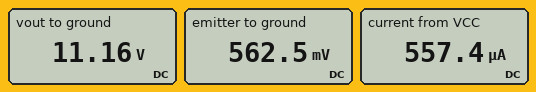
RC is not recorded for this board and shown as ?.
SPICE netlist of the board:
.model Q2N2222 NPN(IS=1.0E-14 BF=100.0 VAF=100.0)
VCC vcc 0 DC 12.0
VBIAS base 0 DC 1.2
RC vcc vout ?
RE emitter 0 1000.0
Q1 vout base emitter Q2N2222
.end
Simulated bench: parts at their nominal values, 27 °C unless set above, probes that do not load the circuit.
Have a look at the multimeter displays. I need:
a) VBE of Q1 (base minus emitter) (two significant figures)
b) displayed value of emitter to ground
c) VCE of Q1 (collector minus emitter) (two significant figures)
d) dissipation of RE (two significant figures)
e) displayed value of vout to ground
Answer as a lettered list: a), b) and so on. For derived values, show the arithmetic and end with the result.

a) 1.2 V - 562.5 mV = 640 mV
b) 562.5 mV
c) 11.16 V - 562.5 mV = 11 V
d) (562.5 mV)^2 / 1 kΩ = 320 µW
e) 11.16 V
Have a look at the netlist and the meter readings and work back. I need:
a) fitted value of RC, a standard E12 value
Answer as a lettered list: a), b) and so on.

a) 1.5 kΩ
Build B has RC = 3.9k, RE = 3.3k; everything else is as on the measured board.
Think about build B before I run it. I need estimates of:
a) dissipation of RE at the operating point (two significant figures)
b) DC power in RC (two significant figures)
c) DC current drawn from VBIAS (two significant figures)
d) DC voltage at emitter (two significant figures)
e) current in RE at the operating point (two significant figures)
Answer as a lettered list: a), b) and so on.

a) 110 µW
b) 120 µW
c) 1.6 µA
d) 590 mV
e) 180 µA
